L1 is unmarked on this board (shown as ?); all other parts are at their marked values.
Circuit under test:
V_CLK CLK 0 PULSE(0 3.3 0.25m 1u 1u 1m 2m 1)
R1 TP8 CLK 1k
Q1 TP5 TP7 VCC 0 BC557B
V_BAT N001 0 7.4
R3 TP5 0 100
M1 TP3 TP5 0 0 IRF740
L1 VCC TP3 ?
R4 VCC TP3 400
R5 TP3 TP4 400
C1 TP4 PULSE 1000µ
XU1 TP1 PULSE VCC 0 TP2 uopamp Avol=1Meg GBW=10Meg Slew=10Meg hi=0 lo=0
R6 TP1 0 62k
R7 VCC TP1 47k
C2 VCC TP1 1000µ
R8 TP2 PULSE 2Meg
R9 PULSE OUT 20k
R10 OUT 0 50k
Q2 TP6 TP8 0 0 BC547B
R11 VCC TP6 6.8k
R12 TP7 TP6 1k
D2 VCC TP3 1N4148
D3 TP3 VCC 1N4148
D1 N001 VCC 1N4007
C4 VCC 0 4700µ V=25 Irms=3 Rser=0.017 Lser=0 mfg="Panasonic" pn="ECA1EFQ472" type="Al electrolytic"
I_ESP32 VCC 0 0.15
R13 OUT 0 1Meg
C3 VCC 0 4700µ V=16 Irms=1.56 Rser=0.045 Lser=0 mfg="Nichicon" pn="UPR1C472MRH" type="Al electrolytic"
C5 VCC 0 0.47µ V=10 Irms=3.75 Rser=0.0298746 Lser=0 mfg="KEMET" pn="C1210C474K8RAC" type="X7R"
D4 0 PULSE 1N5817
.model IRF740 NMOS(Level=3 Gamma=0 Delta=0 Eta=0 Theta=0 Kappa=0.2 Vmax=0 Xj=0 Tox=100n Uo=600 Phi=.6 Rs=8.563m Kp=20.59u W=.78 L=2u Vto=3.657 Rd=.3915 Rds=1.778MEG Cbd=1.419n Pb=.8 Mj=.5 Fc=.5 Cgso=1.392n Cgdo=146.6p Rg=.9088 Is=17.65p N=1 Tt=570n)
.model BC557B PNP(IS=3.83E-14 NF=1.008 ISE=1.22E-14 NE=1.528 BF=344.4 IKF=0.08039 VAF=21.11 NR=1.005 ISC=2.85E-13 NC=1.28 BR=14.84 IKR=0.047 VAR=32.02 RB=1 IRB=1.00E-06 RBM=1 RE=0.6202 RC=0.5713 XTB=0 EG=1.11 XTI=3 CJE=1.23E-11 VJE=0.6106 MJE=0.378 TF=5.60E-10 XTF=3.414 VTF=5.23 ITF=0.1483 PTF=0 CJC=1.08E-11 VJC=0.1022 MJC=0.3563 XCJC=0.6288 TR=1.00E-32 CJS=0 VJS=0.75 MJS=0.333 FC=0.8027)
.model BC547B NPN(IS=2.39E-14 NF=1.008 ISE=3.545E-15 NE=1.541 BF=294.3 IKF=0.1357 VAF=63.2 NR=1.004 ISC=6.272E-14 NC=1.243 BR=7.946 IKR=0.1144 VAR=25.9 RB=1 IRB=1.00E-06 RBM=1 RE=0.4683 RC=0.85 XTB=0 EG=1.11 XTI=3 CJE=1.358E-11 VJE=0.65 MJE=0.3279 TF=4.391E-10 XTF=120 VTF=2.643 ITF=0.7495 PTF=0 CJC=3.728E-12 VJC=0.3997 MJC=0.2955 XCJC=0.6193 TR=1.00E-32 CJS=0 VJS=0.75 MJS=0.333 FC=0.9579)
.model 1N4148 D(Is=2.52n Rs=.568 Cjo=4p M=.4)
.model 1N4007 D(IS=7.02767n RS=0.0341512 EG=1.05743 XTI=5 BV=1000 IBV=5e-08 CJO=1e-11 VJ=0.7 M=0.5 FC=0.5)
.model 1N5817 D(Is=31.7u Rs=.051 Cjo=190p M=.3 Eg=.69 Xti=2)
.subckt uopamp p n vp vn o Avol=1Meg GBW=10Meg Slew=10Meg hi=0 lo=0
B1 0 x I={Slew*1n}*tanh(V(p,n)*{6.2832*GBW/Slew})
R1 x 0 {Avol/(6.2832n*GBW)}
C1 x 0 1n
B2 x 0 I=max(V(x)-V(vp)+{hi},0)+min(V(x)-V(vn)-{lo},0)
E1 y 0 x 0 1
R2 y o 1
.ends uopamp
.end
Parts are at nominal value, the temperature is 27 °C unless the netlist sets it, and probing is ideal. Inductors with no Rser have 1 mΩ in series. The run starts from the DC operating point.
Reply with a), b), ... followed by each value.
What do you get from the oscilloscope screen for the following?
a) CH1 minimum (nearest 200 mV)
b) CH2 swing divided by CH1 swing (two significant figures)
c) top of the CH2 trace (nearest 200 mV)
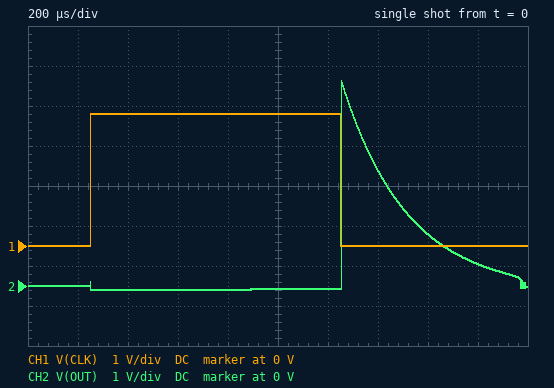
a) 0 V
b) 1.6
c) 5.2 V
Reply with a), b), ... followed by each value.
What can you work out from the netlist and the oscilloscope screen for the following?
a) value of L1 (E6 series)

a) 150 µH
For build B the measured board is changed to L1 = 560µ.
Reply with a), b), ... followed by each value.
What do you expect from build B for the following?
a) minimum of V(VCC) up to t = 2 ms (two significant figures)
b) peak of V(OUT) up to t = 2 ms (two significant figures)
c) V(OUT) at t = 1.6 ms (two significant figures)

a) 6.6 V
b) 2.5 V
c) 1.8 V
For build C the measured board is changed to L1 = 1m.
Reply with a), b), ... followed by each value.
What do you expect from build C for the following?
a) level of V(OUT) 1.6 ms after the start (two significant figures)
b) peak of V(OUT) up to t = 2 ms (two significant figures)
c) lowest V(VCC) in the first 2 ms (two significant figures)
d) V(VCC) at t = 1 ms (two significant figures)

a) 1.4 V
b) 1.6 V
c) 6.6 V
d) 6.7 V
